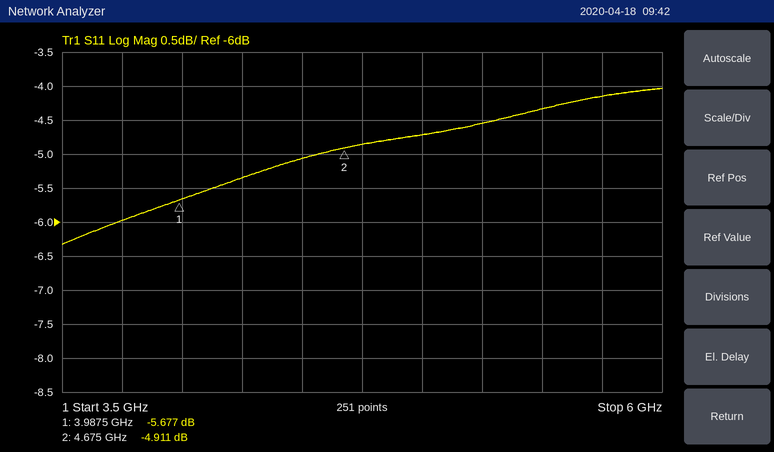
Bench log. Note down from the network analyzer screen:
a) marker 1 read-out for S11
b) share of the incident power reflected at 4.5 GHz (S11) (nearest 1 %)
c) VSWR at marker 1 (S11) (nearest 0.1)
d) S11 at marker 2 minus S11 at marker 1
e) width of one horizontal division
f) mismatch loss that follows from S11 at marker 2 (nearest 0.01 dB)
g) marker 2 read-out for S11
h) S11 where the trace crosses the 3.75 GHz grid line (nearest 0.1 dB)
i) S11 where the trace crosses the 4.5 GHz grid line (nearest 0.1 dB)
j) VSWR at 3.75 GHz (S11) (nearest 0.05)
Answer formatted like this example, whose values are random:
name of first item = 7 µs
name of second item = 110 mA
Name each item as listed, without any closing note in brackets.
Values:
marker 1 read-out for S11 = -5.677 dB
share of the incident power reflected at 4.5 GHz (S11) = 31 %
VSWR at marker 1 (S11) = 3.2
S11 at marker 2 minus S11 at marker 1 = 0.766 dB
width of one horizontal division = 250 MHz
mismatch loss that follows from S11 at marker 2 = 1.69 dB
marker 2 read-out for S11 = -4.911 dB
S11 where the trace crosses the 3.75 GHz grid line = -6.0 dB
S11 where the trace crosses the 4.5 GHz grid line = -5.1 dB
VSWR at 3.75 GHz (S11) = 3.00
